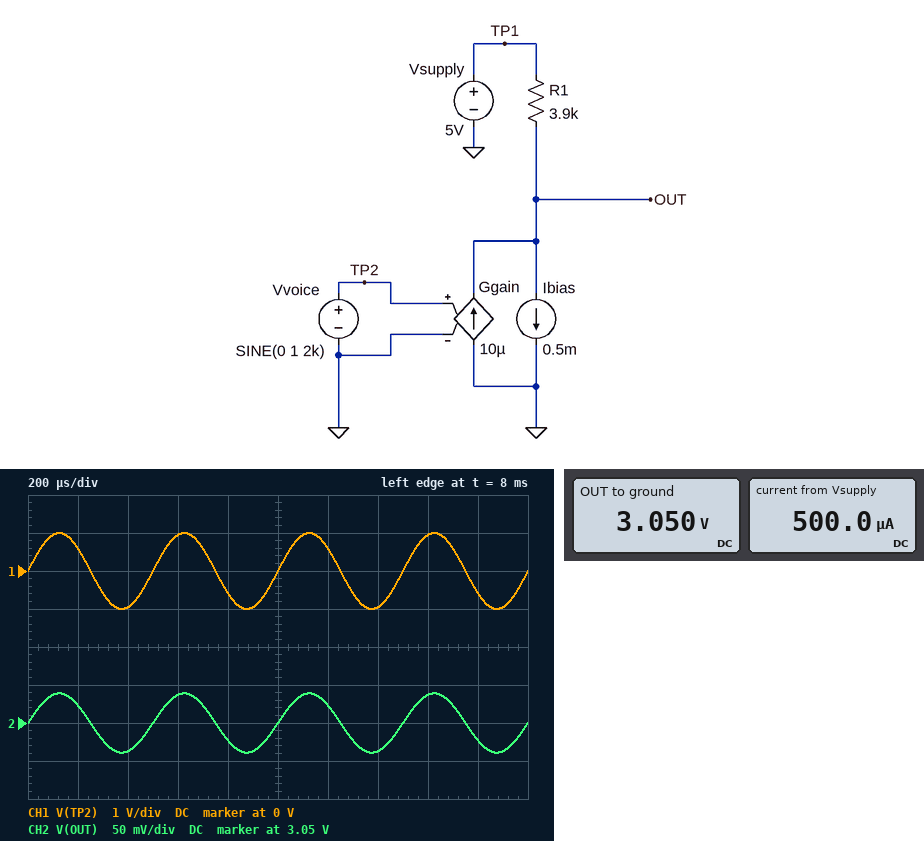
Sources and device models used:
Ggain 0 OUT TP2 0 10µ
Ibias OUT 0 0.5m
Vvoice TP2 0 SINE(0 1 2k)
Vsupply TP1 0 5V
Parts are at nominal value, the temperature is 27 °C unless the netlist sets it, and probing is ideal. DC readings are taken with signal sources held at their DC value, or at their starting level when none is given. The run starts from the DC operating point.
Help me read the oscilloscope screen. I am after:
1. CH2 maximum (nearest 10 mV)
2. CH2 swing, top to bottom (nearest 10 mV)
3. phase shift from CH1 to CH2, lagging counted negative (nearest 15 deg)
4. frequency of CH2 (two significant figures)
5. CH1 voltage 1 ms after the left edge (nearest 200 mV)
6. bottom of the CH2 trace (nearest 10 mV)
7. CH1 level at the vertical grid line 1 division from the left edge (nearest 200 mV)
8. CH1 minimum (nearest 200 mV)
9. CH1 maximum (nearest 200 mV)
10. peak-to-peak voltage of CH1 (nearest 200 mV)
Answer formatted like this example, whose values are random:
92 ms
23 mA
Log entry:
3.09 V
80 mV
0 deg
2.0 kHz
0 V
3.01 V
600 mV
-1.0 V
1.0 V
2.0 V
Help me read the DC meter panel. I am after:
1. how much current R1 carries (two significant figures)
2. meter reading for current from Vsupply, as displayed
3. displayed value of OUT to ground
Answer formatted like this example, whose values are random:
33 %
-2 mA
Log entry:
500 µA
500.0 µA
3.050 V
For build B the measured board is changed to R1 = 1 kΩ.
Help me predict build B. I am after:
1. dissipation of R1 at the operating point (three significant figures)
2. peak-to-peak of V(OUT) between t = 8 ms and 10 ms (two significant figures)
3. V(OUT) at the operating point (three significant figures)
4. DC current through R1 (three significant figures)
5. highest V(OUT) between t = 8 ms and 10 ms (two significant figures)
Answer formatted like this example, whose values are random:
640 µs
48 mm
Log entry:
250 µW
20 mV
4.50 V
500 µA
4.5 V
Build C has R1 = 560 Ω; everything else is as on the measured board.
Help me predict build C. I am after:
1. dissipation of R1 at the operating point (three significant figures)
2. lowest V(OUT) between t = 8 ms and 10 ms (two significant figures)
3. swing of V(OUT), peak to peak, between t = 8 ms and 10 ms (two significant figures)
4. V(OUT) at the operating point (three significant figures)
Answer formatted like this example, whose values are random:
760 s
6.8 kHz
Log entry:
140 µW
4.7 V
11 mV
4.72 V
